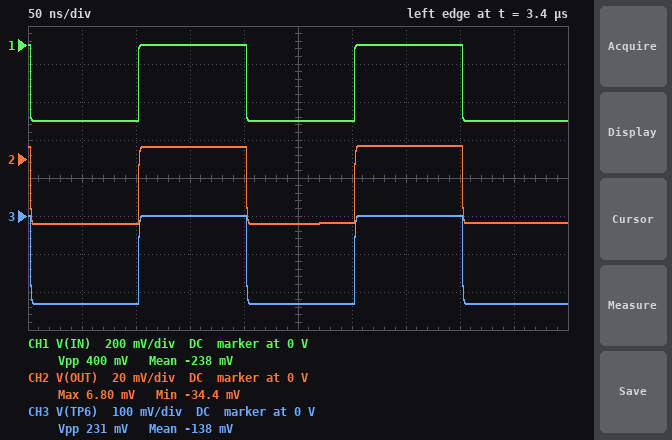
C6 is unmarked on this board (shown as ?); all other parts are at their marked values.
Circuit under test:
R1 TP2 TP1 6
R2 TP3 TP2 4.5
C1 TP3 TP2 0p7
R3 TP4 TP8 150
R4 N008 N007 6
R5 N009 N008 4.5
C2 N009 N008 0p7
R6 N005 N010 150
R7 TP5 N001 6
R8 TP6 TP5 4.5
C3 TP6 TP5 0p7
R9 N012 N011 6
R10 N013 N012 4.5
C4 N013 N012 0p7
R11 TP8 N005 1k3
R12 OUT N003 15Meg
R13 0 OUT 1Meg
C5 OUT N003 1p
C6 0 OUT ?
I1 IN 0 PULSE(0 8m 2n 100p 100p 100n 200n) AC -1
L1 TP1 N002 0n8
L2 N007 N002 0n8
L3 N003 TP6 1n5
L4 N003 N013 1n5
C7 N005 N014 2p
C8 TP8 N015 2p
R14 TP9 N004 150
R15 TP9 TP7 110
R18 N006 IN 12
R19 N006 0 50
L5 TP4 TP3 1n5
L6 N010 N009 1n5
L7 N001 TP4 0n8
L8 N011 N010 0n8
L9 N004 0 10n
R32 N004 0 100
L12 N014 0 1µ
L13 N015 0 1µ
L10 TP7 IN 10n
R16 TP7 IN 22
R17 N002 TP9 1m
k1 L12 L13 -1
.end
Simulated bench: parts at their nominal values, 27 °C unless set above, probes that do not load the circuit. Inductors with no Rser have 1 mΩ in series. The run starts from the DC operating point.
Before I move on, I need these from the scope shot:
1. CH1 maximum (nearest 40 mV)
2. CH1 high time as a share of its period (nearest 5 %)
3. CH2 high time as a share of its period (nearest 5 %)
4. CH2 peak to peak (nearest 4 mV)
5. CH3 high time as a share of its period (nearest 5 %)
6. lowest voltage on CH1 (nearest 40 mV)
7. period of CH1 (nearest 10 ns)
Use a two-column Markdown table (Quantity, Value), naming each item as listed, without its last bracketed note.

| Quantity | Value |
|---|---|
| CH1 maximum | 0 V |
| CH1 high time as a share of its period | 50 % |
| CH2 high time as a share of its period | 50 % |
| CH2 peak to peak | 40 mV |
| CH3 high time as a share of its period | 50 % |
| lowest voltage on CH1 | -400 mV |
| period of CH1 | 200 ns |
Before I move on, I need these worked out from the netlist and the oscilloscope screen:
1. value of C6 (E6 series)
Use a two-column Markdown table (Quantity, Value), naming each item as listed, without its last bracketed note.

| Quantity | Value |
|---|---|
| value of C6 | 4.7 pF |
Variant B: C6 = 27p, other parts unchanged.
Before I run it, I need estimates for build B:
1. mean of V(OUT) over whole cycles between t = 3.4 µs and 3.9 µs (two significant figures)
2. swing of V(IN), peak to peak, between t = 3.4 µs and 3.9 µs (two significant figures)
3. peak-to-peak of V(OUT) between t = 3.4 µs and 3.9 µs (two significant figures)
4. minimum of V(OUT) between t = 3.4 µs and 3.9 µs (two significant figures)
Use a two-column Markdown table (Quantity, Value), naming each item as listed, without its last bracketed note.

| Quantity | Value |
|---|---|
| mean of V(OUT) over whole cycles between t = 3.4 µs and 3.9 µs | -4.5 mV |
| swing of V(IN), peak to peak, between t = 3.4 µs and 3.9 µs | 400 mV |
| peak-to-peak of V(OUT) between t = 3.4 µs and 3.9 µs | 8.3 mV |
| minimum of V(OUT) between t = 3.4 µs and 3.9 µs | -8.7 mV |
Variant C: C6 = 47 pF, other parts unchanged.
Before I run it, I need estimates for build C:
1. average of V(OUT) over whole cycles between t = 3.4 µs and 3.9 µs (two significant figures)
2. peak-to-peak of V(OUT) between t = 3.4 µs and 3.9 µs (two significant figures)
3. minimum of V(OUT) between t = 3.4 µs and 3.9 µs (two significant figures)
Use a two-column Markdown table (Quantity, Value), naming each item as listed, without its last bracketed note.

| Quantity | Value |
|---|---|
| average of V(OUT) over whole cycles between t = 3.4 µs and 3.9 µs | -2.8 mV |
| peak-to-peak of V(OUT) between t = 3.4 µs and 3.9 µs | 4.9 mV |
| minimum of V(OUT) between t = 3.4 µs and 3.9 µs | -5.2 mV |
